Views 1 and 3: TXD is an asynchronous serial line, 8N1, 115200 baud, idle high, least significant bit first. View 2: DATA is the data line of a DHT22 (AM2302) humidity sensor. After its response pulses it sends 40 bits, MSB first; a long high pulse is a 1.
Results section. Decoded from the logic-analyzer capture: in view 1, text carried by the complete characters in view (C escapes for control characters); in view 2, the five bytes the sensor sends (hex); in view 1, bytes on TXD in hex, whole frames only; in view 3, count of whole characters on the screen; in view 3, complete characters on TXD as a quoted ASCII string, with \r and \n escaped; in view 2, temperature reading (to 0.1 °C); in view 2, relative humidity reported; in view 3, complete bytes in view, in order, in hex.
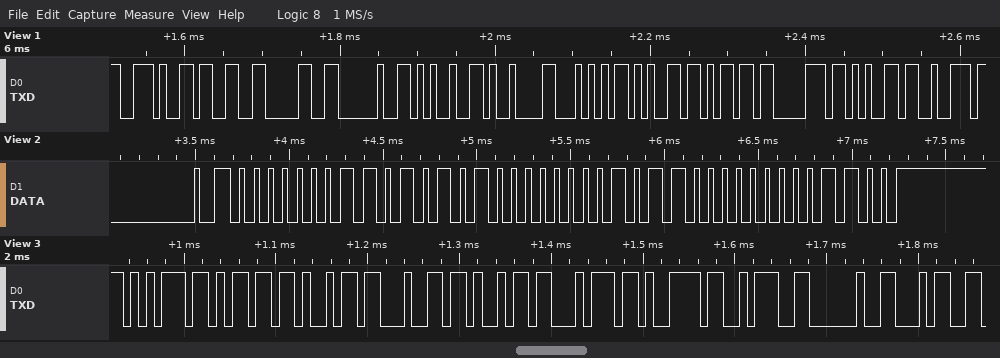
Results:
".30 %\tTemper"
01 AA 01 60 0C
2E 33 30 20 25 09 54 65 6D 70 65 72
10
"umidity: 4"
35.2 °C
42.6 %
75 6D 69 64 69 74 79 3A 20 34
